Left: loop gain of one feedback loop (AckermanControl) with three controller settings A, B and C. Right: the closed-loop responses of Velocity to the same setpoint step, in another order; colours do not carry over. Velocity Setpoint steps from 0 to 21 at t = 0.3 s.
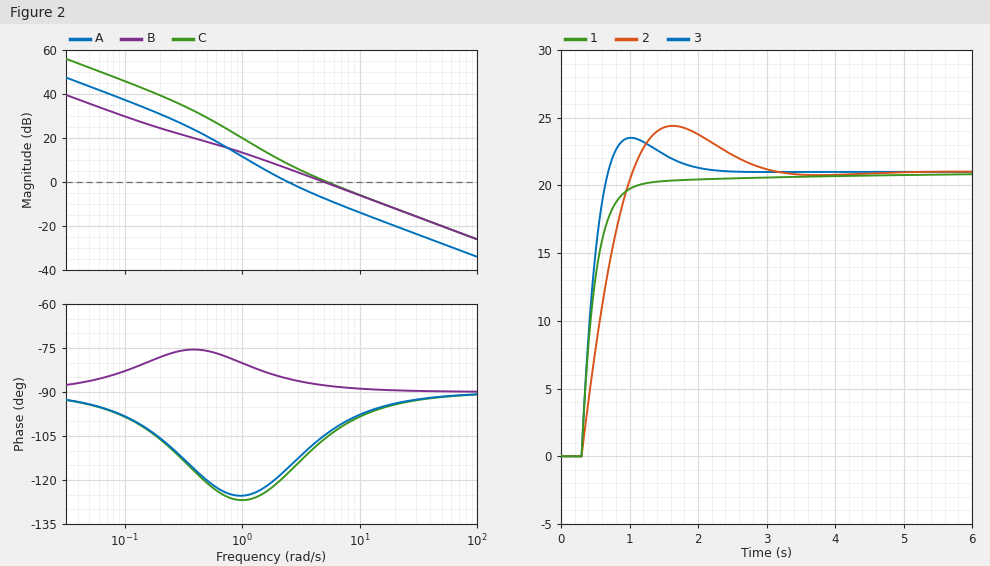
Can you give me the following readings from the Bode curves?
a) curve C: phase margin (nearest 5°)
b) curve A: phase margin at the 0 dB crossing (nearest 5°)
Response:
75°
65°
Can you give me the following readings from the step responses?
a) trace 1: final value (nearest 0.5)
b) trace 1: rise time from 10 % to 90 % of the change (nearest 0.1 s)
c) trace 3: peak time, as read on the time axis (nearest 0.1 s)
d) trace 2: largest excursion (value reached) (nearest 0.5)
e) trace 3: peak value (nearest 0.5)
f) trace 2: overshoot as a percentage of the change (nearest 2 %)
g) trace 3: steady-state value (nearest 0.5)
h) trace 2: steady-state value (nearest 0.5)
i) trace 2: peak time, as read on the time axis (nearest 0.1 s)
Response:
21.0
0.5 s
1.0 s
24.5
23.5
16 %
21.0
21.0
1.6 s
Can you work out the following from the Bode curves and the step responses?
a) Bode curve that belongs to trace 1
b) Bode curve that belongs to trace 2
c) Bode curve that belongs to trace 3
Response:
B
A
C
